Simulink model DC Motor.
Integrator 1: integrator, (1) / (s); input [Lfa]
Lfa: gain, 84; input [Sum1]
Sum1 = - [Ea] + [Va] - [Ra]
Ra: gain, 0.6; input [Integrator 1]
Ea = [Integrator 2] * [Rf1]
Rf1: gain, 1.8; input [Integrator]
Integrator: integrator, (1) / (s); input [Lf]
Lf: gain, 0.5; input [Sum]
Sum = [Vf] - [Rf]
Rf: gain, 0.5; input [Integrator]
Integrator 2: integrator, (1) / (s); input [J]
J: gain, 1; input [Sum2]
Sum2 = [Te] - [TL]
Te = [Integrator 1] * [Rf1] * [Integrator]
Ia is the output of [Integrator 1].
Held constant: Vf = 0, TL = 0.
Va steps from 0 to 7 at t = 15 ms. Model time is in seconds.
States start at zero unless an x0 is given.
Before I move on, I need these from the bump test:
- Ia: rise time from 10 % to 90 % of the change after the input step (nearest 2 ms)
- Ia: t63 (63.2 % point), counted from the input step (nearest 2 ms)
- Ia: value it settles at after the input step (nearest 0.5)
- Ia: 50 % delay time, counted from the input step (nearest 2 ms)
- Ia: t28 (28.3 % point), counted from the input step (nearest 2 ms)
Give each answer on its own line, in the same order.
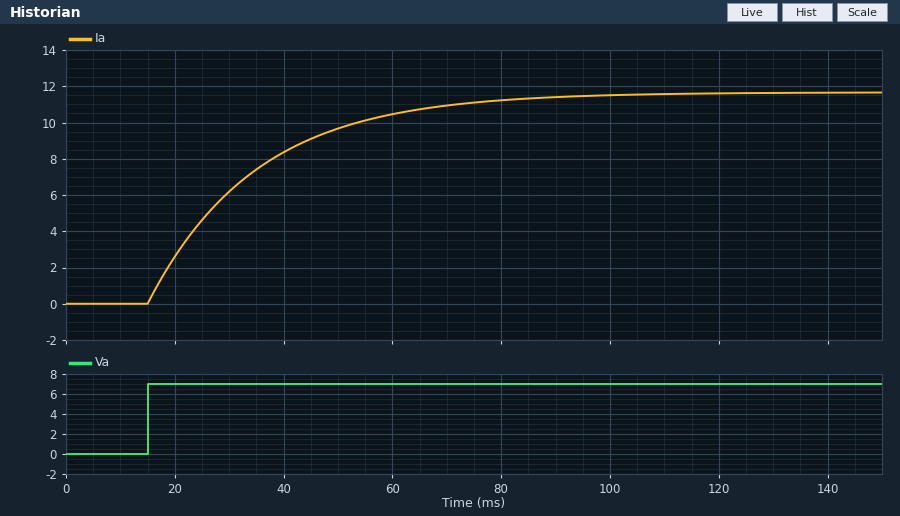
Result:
44 ms
20 ms
11.5
14 ms
6 ms
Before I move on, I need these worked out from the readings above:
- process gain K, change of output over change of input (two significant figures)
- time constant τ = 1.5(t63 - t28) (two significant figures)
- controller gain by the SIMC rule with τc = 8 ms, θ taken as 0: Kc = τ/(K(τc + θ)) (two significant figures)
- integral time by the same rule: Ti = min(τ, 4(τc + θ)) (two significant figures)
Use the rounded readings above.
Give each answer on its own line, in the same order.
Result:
1.6
21 ms
1.6
21 ms
